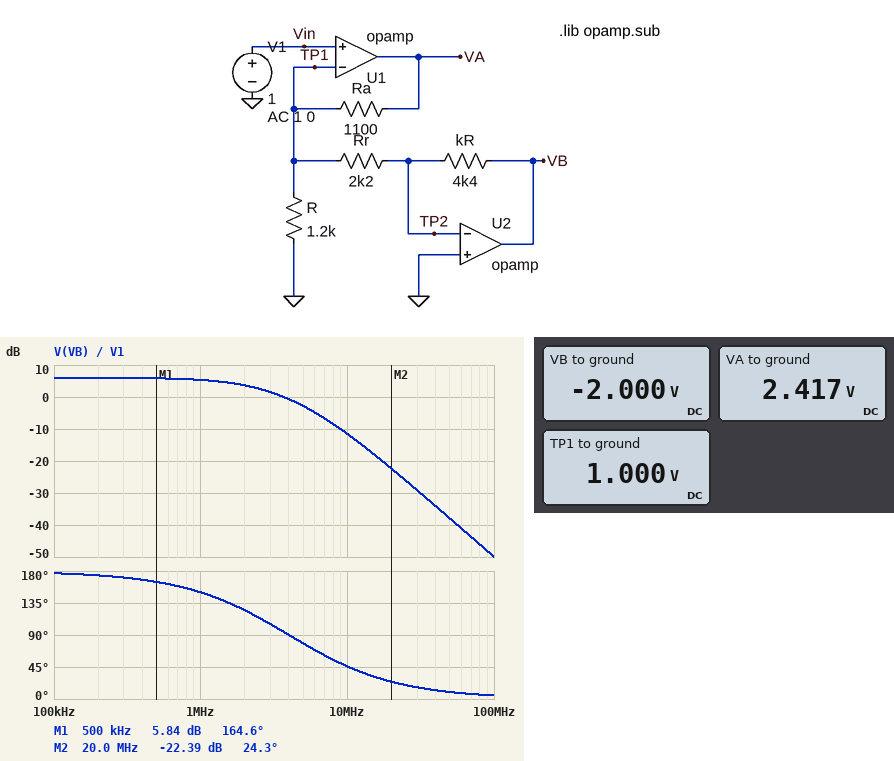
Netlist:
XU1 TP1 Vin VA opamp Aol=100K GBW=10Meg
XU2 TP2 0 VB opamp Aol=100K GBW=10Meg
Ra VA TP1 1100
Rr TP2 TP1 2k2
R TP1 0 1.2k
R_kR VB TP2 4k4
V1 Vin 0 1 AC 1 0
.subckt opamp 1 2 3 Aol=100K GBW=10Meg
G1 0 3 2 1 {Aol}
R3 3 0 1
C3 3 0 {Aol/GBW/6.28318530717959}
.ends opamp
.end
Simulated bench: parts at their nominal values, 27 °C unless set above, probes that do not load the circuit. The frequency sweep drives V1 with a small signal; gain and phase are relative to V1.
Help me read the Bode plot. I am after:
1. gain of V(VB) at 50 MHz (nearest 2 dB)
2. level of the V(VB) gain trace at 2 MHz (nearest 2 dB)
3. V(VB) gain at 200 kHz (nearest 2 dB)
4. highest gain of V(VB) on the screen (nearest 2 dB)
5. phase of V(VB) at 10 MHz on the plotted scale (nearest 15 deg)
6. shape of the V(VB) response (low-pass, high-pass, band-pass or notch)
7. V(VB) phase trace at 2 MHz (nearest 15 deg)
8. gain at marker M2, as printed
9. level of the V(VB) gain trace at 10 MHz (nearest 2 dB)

-38 dB
4 dB
6 dB
6 dB
45 deg
low-pass
120 deg
-22.39 dB
-12 dB
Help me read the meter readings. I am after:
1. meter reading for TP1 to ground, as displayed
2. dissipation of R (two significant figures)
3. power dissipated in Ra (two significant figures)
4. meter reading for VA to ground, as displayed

1.000 V
830 µW
1.8 mW
2.417 V
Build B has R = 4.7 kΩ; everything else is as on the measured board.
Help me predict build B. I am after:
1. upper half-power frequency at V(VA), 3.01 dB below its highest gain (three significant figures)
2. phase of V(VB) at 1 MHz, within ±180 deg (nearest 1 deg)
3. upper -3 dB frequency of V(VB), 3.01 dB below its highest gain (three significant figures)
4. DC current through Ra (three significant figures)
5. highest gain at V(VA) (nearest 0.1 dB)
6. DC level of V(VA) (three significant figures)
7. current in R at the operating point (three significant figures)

4.27 MHz
154 deg
2.57 MHz
667 µA
4.8 dB
1.73 V
213 µA
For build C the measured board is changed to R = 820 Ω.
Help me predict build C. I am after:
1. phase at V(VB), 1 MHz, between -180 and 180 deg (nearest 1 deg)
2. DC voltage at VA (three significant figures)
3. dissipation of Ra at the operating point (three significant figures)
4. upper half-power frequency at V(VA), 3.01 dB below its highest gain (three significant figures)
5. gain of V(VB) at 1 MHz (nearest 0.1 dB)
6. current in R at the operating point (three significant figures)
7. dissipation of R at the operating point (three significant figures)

148 deg
2.84 V
3.08 mW
3.09 MHz
5.2 dB
1.22 mA
1.22 mW
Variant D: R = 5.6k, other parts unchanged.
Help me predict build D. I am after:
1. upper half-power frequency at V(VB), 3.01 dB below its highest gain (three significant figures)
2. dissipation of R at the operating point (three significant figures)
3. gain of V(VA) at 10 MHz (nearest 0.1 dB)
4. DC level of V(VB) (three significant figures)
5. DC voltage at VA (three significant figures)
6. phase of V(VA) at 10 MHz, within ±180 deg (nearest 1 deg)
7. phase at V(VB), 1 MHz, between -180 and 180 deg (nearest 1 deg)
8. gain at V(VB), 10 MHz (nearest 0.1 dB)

2.58 MHz
179 µW
-2.1 dB
-2.00 V
1.70 V
-56 deg
154 deg
-9.0 dB
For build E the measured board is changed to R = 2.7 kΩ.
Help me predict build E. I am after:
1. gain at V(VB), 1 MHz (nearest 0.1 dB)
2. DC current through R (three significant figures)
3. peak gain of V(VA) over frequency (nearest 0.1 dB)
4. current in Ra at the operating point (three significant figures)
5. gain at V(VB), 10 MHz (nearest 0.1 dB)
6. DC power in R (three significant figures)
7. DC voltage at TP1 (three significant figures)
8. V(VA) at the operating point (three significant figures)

5.4 dB
370 µA
5.6 dB
825 µA
-9.8 dB
370 µW
1.00 V
1.91 V
